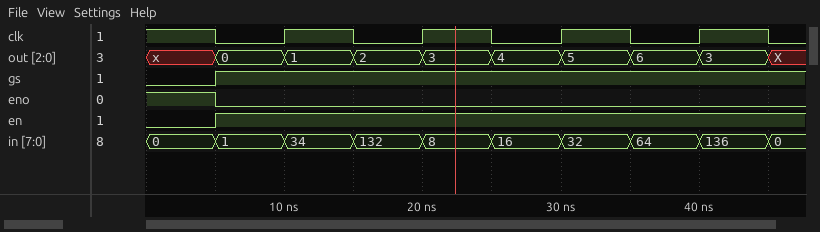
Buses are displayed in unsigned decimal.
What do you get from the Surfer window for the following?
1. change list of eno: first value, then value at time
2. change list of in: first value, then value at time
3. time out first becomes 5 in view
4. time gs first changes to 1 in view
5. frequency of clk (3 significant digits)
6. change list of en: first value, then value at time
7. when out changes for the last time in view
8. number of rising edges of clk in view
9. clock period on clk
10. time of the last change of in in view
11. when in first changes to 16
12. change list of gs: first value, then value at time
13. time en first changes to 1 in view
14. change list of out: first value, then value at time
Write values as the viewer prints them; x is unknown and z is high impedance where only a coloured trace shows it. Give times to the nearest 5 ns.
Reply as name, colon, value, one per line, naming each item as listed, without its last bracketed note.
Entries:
change list of eno: first value, then value at time: 1, 0 at 5 ns
change list of in: first value, then value at time: 0, 1 at 5 ns, 34 at 10 ns, 132 at 15 ns, 8 at 20 ns, 16 at 25 ns, 32 at 30 ns, 64 at 35 ns, 136 at 40 ns, 0 at 45 ns
time out first becomes 5 in view: 30 ns
time gs first changes to 1 in view: 5 ns
frequency of clk: 100 MHz
change list of en: first value, then value at time: 0, 1 at 5 ns
when out changes for the last time in view: 45 ns
number of rising edges of clk in view: 4
clock period on clk: 10 ns
time of the last change of in in view: 45 ns
when in first changes to 16: 25 ns
change list of gs: first value, then value at time: 0, 1 at 5 ns
time en first changes to 1 in view: 5 ns
change list of out: first value, then value at time: x, 0 at 5 ns, 1 at 10 ns, 2 at 15 ns, 3 at 20 ns, 4 at 25 ns, 5 at 30 ns, 6 at 35 ns, 3 at 40 ns, X at 45 ns
